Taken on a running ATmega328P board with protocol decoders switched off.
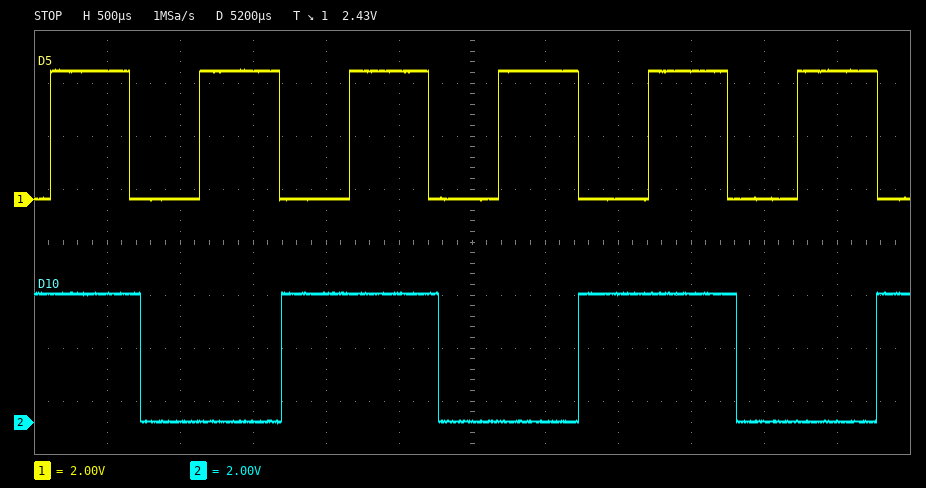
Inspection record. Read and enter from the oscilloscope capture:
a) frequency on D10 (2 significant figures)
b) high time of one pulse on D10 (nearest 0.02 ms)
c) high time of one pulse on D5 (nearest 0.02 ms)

490 Hz
1.08 ms
0.54 ms
